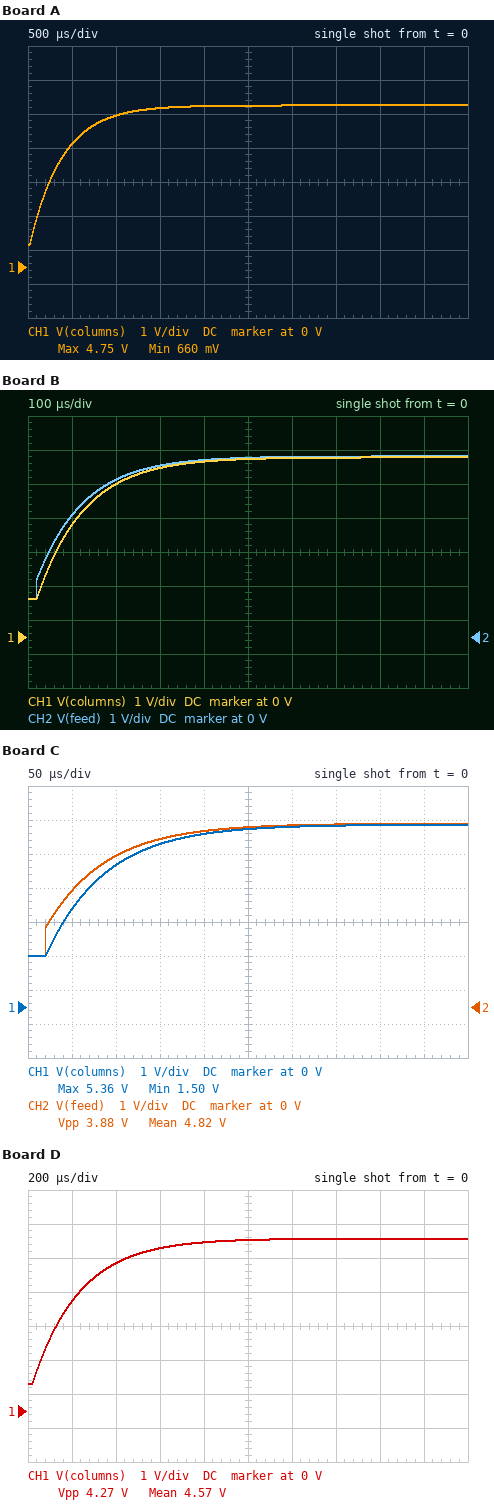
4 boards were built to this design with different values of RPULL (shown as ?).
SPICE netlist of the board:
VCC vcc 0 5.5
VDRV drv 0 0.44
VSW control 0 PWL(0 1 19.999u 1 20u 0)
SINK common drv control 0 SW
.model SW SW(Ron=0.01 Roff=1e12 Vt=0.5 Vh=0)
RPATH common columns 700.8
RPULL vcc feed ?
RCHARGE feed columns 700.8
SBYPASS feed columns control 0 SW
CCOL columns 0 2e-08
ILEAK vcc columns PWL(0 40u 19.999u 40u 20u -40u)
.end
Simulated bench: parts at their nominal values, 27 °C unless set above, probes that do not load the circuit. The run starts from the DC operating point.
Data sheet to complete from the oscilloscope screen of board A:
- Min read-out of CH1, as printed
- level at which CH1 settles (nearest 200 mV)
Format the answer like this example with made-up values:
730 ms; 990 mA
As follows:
660 mV; 4.8 V
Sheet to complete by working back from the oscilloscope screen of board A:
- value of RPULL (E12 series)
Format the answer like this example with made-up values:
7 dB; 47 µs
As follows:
18 kΩ
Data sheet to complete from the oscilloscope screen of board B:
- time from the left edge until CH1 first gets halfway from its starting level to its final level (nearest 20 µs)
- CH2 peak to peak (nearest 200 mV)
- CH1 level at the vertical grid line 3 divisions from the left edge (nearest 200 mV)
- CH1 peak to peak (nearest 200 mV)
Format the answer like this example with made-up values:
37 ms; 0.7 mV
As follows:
100 µs; 4.2 V; 5.0 V; 4.2 V
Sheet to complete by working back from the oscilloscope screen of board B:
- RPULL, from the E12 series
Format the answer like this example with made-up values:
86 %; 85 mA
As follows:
4.7 kΩ
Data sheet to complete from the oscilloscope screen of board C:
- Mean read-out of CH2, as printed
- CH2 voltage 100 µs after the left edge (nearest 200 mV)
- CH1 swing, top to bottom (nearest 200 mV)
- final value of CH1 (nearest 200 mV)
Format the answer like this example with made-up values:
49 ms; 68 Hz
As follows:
4.82 V; 4.4 V; 3.8 V; 5.4 V
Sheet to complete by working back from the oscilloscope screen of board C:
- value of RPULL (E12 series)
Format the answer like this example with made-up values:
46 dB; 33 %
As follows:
2.7 kΩ
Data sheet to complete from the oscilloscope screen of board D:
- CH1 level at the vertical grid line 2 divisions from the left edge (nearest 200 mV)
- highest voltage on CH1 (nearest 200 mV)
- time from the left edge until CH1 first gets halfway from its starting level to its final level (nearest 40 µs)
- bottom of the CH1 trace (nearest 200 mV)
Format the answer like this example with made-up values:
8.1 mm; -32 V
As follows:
4.4 V; 5.0 V; 160 µs; 800 mV
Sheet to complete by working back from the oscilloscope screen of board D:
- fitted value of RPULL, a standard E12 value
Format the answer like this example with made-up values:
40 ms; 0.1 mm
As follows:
10 kΩ
